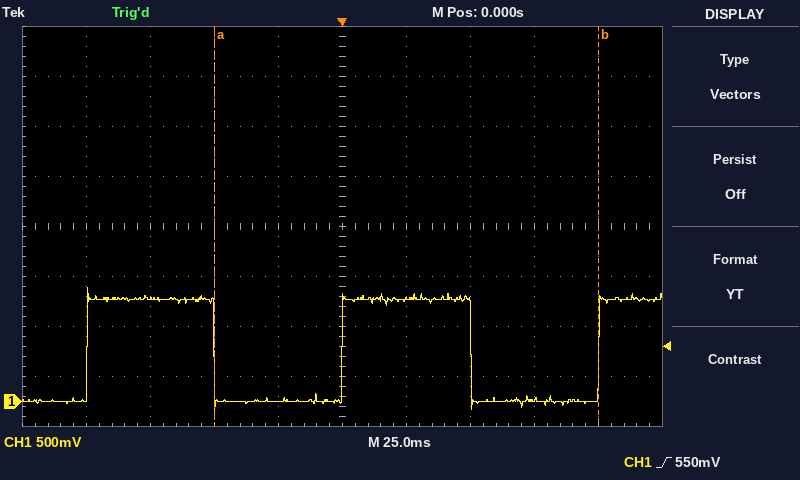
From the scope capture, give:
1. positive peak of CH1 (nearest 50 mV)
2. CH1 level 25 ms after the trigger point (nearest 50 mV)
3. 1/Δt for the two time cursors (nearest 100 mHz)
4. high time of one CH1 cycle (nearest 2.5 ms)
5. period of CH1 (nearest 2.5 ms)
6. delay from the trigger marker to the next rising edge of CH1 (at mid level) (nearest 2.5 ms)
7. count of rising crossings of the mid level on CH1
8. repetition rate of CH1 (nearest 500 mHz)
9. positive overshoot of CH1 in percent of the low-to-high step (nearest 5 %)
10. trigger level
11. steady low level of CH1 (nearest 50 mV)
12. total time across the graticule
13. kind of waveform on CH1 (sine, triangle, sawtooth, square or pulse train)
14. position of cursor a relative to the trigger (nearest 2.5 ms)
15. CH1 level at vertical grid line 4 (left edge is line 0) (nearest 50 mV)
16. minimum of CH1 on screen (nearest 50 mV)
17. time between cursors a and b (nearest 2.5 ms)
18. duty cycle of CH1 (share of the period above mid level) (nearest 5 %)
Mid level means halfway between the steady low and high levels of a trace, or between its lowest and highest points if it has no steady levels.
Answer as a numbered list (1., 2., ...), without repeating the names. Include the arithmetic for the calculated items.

1. 1.15 V
2. 1.00 V
3. 1 / 150.0 ms ≈ 6.7 Hz
4. 50.0 ms
5. 100.0 ms
6. 100.0 ms
7. 3
8. 1 / 100.0 ms ≈ 10.0 Hz
9. 10 %
10. 550 mV
11. 0 mV
12. 250 ms
13. square
14. -50.0 ms
15. 0 mV
16. -100 mV
17. 150.0 ms
18. 50.0 ms / 100.0 ms ≈ 50 %
